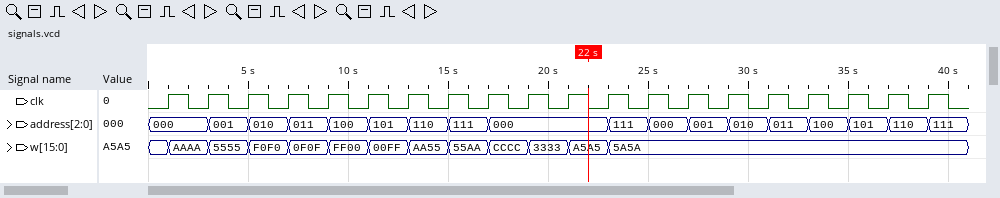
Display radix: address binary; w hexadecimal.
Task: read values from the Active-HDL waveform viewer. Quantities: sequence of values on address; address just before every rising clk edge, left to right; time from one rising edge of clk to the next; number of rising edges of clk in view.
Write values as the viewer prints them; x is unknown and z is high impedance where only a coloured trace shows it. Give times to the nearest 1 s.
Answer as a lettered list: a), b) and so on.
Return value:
a) 000, 001, 010, 011, 100, 101, 110, 111, 000, 111, 000, 001, 010, 011, 100, 101, 110, 111
b) 000, 000, 001, 010, 011, 100, 101, 110, 111, 000, 000, 000, 111, 000, 001, 010, 011, 100, 101, 110
c) 2 s
d) 20
